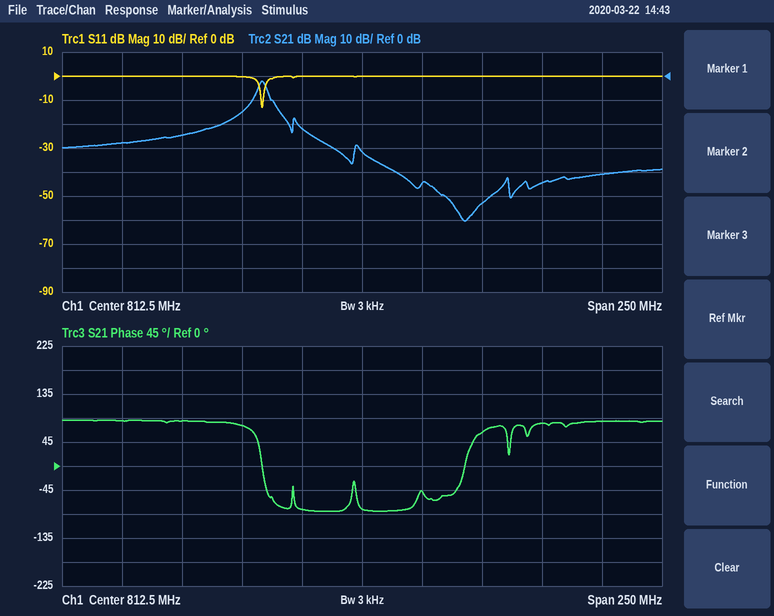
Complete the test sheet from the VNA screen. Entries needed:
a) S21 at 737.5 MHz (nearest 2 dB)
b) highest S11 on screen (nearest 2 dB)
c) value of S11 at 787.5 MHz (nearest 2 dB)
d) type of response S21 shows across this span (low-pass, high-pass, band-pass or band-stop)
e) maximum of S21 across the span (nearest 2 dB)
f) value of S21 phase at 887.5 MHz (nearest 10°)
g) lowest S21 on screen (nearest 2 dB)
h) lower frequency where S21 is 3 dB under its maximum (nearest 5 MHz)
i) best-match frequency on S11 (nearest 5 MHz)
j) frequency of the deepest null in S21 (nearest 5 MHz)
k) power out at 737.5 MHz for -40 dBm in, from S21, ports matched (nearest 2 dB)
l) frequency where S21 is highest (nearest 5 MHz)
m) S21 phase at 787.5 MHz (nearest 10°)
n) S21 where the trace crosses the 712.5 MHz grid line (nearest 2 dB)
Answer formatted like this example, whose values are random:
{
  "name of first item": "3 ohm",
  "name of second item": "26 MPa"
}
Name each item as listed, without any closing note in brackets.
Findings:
{
  "S21 at 737.5 MHz": "-24 dB",
  "highest S11 on screen": "0 dB",
  "value of S11 at 787.5 MHz": "0 dB",
  "type of response S21 shows across this span": "band-pass",
  "maximum of S21 across the span": "-2 dB",
  "value of S21 phase at 887.5 MHz": "80°",
  "lowest S21 on screen": "-60 dB",
  "lower frequency where S21 is 3 dB under its maximum": "770 MHz",
  "best-match frequency on S11": "770 MHz",
  "frequency of the deepest null in S21": "855 MHz",
  "power out at 737.5 MHz for -40 dBm in, from S21, ports matched": "-64 dBm",
  "frequency where S21 is highest": "770 MHz",
  "S21 phase at 787.5 MHz": "-80°",
  "S21 where the trace crosses the 712.5 MHz grid line": "-28 dB"
}
